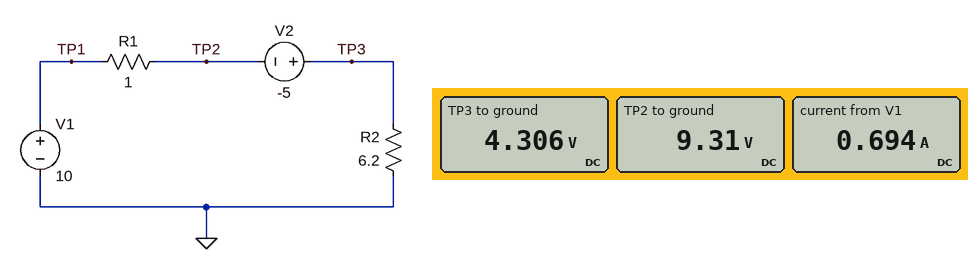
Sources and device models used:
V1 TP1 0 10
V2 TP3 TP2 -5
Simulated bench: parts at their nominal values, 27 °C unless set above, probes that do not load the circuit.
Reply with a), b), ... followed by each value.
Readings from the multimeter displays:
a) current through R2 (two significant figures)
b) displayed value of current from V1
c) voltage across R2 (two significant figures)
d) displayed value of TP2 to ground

a) 690 mA
b) 0.694 A
c) 4.3 V
d) 9.31 V
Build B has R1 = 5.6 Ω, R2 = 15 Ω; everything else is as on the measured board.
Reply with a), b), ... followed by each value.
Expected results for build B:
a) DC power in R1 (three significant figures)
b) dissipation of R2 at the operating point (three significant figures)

a) 330 mW
b) 884 mW
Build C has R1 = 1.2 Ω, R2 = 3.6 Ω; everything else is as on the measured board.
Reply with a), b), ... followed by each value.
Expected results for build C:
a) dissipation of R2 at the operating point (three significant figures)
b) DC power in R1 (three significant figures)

a) 3.91 W
b) 1.30 W
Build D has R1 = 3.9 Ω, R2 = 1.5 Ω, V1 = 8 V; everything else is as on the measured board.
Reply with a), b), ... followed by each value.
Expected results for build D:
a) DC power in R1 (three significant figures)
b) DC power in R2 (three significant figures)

a) 1.20 W
b) 463 mW
